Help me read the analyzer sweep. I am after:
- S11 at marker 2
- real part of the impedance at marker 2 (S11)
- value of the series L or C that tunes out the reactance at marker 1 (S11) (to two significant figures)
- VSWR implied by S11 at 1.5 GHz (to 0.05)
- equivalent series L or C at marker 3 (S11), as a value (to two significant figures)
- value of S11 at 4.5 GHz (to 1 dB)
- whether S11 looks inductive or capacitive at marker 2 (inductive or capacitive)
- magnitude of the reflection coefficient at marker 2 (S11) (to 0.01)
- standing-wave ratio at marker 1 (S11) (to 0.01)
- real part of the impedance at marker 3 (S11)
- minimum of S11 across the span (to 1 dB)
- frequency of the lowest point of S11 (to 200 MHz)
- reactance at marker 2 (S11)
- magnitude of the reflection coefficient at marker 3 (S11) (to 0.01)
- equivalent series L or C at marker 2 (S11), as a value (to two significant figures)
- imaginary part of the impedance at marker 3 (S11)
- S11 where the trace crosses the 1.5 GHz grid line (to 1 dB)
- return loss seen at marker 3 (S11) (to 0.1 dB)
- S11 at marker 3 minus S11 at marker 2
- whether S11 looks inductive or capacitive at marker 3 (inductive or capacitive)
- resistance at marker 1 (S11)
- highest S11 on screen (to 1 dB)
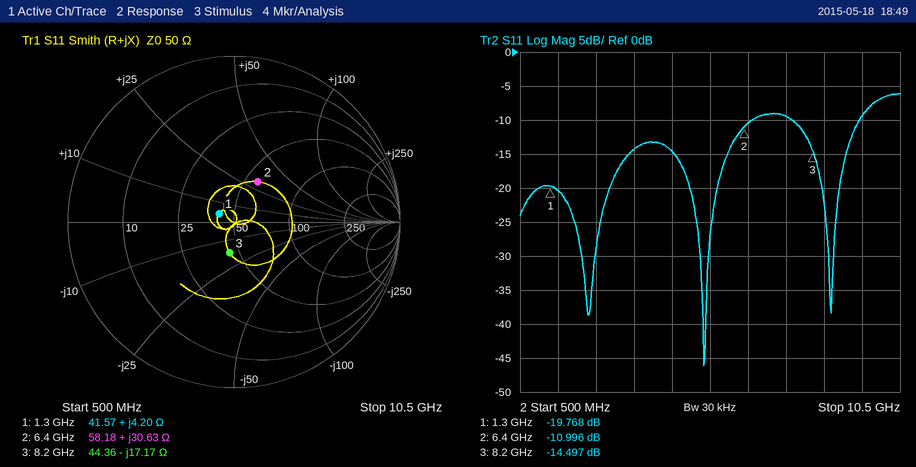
-10.996 dB
58.18 Ω
29 pF
1.20
1.1 pF
-15 dB
inductive
0.28
1.23
44.36 Ω
-46 dB
5.4 GHz
+30.63 Ω
0.19
760 pH
-17.17 Ω
-20 dB
14.5 dB
-3.501 dB
capacitive
41.57 Ω
-6 dB
